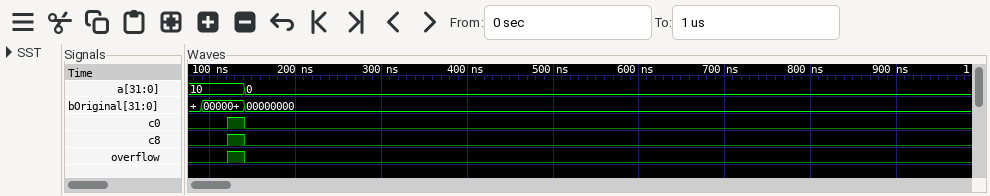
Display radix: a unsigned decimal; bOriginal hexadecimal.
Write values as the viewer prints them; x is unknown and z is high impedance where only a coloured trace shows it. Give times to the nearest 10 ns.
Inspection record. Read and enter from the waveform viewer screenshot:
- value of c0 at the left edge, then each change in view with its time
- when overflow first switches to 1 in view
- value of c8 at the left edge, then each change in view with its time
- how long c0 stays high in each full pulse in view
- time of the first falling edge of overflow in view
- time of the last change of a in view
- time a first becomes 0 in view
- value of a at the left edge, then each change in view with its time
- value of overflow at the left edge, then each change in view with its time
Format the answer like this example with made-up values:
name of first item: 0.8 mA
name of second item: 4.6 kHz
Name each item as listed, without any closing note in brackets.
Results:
value of c0 at the left edge, then each change in view with its time: 0, 1 at 120 ns, 0 at 140 ns
when overflow first switches to 1 in view: 120 ns
value of c8 at the left edge, then each change in view with its time: 0, 1 at 120 ns, 0 at 140 ns
how long c0 stays high in each full pulse in view: 20 ns
time of the first falling edge of overflow in view: 140 ns
time of the last change of a in view: 140 ns
time a first becomes 0 in view: 140 ns
value of a at the left edge, then each change in view with its time: 10, 0 at 140 ns
value of overflow at the left edge, then each change in view with its time: 0, 1 at 120 ns, 0 at 140 ns
